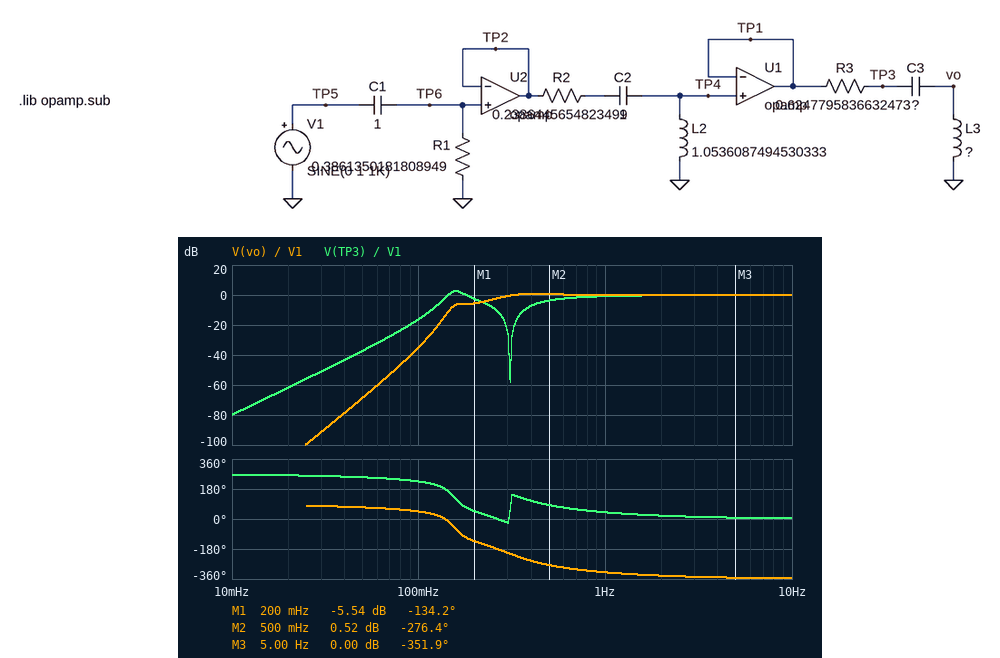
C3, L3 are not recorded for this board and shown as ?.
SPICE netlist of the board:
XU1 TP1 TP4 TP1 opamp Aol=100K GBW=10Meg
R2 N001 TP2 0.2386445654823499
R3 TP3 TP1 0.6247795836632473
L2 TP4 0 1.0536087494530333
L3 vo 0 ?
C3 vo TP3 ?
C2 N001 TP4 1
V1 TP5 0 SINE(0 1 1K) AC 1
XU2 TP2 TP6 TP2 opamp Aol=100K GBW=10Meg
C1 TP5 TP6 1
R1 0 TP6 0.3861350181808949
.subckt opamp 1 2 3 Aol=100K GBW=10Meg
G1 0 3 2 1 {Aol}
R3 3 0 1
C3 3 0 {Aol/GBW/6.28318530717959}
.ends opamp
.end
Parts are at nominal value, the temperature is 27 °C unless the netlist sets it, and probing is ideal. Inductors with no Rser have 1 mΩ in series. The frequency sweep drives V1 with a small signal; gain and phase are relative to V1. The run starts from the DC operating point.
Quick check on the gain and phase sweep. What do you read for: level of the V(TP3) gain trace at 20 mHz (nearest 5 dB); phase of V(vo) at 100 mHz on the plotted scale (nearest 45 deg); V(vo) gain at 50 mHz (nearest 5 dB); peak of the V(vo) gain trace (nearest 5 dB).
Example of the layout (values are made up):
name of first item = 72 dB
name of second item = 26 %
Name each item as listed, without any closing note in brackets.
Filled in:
level of the V(TP3) gain trace at 20 mHz = -60 dB
phase of V(vo) at 100 mHz on the plotted scale = 45 deg
V(vo) gain at 50 mHz = -70 dB
peak of the V(vo) gain trace = 0 dB
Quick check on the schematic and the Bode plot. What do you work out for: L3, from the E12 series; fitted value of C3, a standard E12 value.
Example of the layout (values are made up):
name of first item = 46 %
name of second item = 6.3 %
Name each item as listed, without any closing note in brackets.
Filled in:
L3, from the E12 series = 390 mH
fitted value of C3, a standard E12 value = 680 mF
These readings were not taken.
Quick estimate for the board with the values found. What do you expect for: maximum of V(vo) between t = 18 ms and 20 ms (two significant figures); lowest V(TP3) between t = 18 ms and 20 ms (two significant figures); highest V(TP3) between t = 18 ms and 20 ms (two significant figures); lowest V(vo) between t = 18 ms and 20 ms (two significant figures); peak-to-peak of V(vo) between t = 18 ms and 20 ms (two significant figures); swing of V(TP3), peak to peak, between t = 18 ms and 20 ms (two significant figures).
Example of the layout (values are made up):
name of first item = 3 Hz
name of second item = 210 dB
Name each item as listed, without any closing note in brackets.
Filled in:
maximum of V(vo) between t = 18 ms and 20 ms = 1.0 V
lowest V(TP3) between t = 18 ms and 20 ms = -1.0 V
highest V(TP3) between t = 18 ms and 20 ms = 1.0 V
lowest V(vo) between t = 18 ms and 20 ms = -1.0 V
peak-to-peak of V(vo) between t = 18 ms and 20 ms = 2.0 V
swing of V(TP3), peak to peak, between t = 18 ms and 20 ms = 2.0 V
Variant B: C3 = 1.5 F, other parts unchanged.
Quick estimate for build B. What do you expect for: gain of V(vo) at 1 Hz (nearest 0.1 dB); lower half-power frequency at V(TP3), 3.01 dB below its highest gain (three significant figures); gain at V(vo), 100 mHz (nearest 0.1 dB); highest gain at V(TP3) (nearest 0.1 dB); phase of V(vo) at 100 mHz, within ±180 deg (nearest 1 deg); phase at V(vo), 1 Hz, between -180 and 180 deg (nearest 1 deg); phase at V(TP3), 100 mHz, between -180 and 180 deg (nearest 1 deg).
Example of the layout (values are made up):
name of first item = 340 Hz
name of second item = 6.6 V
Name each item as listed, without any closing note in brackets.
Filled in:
gain of V(vo) at 1 Hz = -0.4 dB
lower half-power frequency at V(TP3), 3.01 dB below its highest gain = 481 mHz
gain at V(vo), 100 mHz = -28.2 dB
highest gain at V(TP3) = 0 dB
phase of V(vo) at 100 mHz, within ±180 deg = 24 deg
phase at V(vo), 1 Hz, between -180 and 180 deg = 39 deg
phase at V(TP3), 100 mHz, between -180 and 180 deg = -156 deg
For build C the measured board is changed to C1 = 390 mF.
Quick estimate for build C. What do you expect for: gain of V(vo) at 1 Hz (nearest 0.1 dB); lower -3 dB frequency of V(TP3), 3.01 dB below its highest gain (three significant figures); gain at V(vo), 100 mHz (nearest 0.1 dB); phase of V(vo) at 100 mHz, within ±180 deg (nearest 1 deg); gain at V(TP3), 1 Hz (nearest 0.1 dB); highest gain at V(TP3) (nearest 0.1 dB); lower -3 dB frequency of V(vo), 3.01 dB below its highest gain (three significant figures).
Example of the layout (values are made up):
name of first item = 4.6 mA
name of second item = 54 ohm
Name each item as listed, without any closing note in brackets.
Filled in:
gain of V(vo) at 1 Hz = -2.5 dB
lower -3 dB frequency of V(TP3), 3.01 dB below its highest gain = 1.08 Hz
gain at V(vo), 100 mHz = -42.8 dB
phase of V(vo) at 100 mHz, within ±180 deg = 53 deg
gain at V(TP3), 1 Hz = -3.4 dB
highest gain at V(TP3) = 0 dB
lower -3 dB frequency of V(vo), 3.01 dB below its highest gain = 856 mHz
